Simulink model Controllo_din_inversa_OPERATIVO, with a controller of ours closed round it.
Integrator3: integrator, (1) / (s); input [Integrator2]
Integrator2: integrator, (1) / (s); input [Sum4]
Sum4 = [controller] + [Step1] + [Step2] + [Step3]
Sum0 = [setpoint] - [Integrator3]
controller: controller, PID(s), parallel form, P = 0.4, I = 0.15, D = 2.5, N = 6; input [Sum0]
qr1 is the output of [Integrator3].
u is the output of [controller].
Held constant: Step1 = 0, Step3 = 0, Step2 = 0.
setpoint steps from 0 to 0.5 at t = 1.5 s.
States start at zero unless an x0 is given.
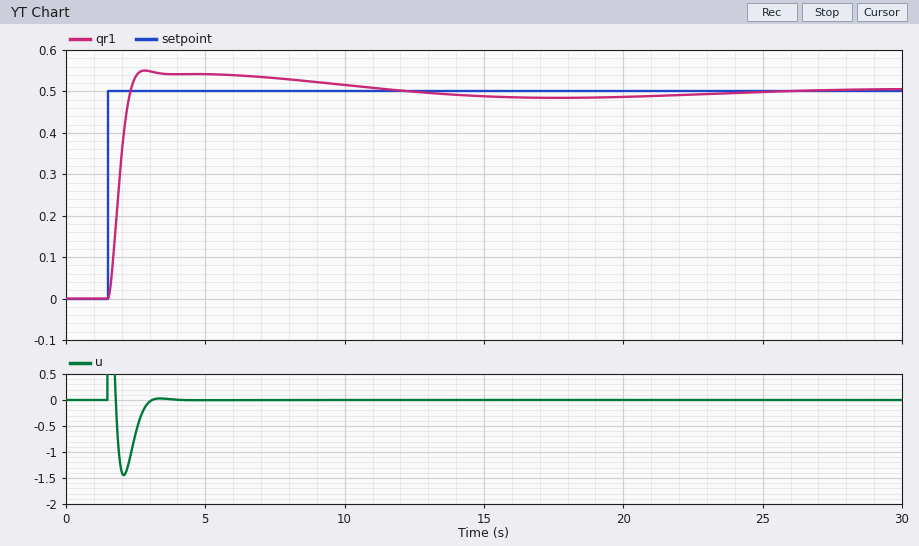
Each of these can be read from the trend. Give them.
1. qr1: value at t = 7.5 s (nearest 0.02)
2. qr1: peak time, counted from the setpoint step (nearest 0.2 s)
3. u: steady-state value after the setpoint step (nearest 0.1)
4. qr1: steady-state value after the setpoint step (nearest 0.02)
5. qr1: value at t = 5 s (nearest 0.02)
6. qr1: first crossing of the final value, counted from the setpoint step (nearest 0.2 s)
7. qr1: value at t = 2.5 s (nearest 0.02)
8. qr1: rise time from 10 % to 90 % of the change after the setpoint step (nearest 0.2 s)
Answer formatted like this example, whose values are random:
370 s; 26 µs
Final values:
0.54; 1.4 s; 0.0; 0.50; 0.54; 0.8 s; 0.54; 0.6 s
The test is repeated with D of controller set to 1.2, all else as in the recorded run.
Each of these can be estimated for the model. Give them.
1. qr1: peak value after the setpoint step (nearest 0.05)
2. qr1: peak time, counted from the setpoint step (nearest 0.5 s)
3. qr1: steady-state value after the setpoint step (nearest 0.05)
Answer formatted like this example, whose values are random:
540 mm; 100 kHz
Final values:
0.65; 3.0 s; 0.50
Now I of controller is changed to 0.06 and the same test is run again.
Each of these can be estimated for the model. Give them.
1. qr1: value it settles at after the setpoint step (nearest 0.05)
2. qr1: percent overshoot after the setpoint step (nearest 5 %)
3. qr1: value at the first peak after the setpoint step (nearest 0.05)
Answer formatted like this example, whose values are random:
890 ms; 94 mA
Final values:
0.50; 10 %; 0.55
